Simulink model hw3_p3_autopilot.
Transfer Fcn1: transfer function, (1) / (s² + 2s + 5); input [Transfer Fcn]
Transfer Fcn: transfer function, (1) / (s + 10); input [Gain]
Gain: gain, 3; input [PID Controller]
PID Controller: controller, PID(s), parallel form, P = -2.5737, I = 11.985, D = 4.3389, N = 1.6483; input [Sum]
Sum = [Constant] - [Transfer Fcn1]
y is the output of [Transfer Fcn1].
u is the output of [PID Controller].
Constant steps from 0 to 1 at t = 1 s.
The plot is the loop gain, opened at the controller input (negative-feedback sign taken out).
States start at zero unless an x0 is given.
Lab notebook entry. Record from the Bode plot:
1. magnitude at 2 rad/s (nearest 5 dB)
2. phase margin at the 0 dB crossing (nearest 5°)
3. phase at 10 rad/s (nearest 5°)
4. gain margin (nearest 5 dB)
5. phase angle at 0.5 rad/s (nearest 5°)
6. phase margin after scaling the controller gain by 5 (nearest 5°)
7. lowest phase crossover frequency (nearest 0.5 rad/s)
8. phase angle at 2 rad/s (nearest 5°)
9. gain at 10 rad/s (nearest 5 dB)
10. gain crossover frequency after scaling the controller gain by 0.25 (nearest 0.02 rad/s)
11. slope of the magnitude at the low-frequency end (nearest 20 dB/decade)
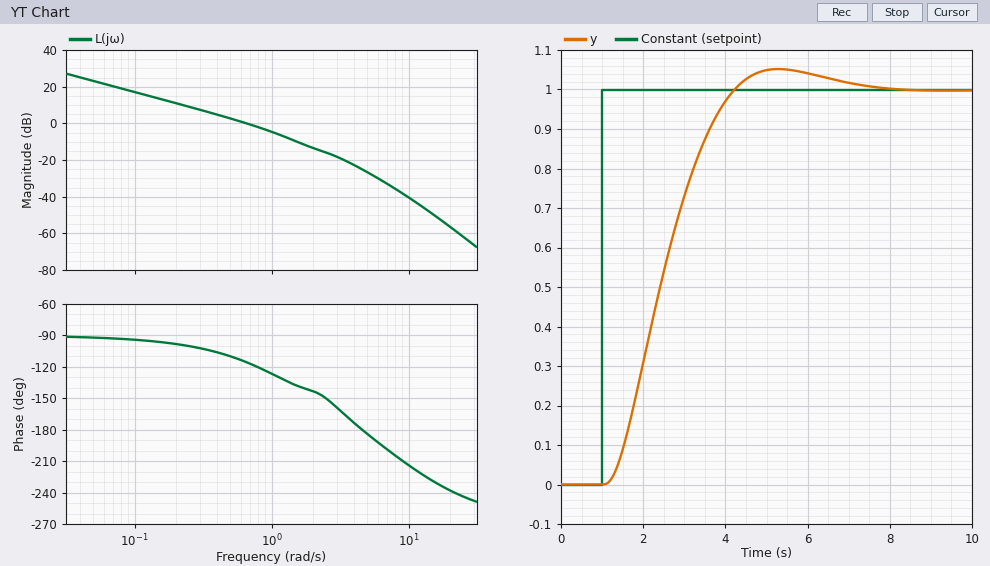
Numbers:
-15 dB
65°
-215°
25 dB
-110°
35°
4.5 rad/s
-145°
-40 dB
0.18 rad/s
-20 dB/decade
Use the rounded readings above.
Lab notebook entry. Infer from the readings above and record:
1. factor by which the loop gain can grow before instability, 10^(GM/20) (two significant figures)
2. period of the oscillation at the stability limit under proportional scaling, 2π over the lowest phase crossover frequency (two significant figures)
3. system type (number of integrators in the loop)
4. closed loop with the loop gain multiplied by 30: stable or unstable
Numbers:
18
1.4 s
1
unstable
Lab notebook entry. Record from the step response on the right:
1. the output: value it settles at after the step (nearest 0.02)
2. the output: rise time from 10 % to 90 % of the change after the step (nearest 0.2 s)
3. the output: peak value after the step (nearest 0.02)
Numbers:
1.00
2.0 s
1.06
